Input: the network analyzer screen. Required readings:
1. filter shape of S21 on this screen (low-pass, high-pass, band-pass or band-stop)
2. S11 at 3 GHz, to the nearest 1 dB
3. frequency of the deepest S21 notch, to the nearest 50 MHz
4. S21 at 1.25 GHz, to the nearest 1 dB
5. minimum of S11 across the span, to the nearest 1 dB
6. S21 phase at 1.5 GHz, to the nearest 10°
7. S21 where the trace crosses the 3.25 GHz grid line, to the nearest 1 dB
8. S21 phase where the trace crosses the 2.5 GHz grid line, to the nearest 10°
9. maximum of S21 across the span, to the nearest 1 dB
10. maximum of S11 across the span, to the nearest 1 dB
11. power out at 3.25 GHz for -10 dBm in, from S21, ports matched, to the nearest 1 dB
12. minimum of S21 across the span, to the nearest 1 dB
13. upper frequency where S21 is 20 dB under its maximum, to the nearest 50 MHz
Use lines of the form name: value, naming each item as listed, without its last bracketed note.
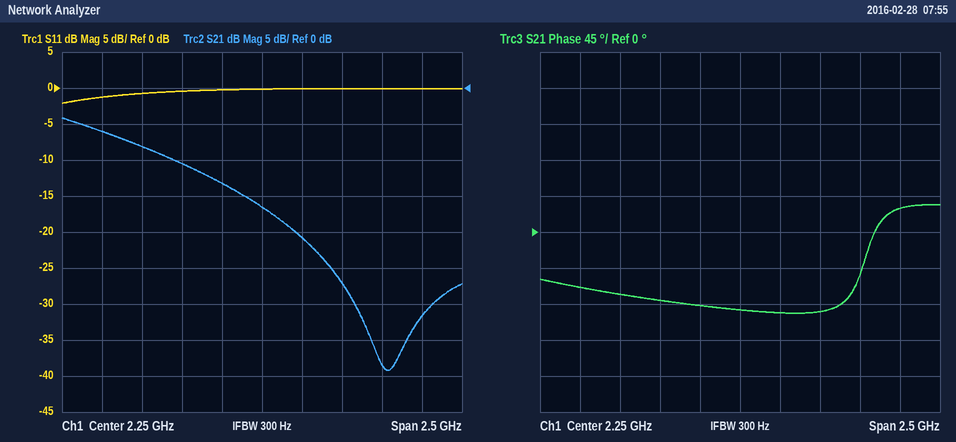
filter shape of S21 on this screen: low-pass
S11 at 3 GHz, to the nearest 1 dB: 0 dB
frequency of the deepest S21 notch, to the nearest 50 MHz: 3.05 GHz
S21 at 1.25 GHz, to the nearest 1 dB: -6 dB
minimum of S11 across the span, to the nearest 1 dB: -2 dB
S21 phase at 1.5 GHz, to the nearest 10°: -80°
S21 where the trace crosses the 3.25 GHz grid line, to the nearest 1 dB: -32 dB
S21 phase where the trace crosses the 2.5 GHz grid line, to the nearest 10°: -100°
maximum of S21 across the span, to the nearest 1 dB: -4 dB
maximum of S11 across the span, to the nearest 1 dB: 0 dB
power out at 3.25 GHz for -10 dBm in, from S21, ports matched, to the nearest 1 dB: -42 dBm
minimum of S21 across the span, to the nearest 1 dB: -39 dB
upper frequency where S21 is 20 dB under its maximum, to the nearest 50 MHz: 2.65 GHz
